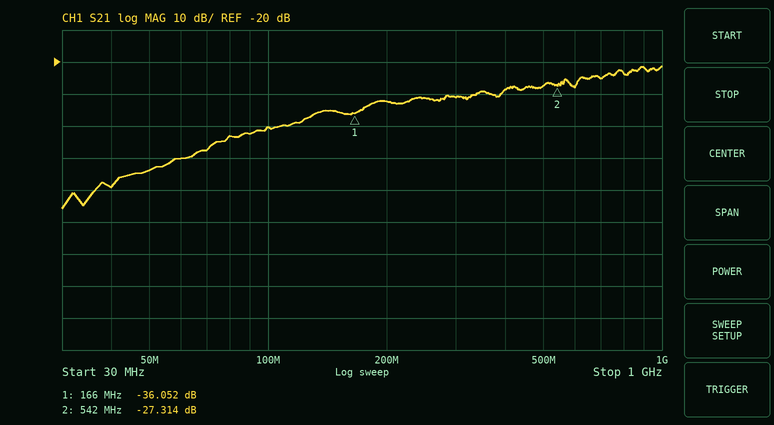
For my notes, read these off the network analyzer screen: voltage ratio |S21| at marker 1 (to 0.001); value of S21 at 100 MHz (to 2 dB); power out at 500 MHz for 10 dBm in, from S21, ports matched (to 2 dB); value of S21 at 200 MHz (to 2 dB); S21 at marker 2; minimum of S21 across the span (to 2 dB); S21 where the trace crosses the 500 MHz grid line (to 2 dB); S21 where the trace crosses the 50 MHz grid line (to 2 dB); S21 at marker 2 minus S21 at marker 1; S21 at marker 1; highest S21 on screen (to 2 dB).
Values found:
0.016
-40 dB
-18 dBm
-32 dB
-27.314 dB
-66 dB
-28 dB
-54 dB
8.738 dB
-36.052 dB
-22 dB
